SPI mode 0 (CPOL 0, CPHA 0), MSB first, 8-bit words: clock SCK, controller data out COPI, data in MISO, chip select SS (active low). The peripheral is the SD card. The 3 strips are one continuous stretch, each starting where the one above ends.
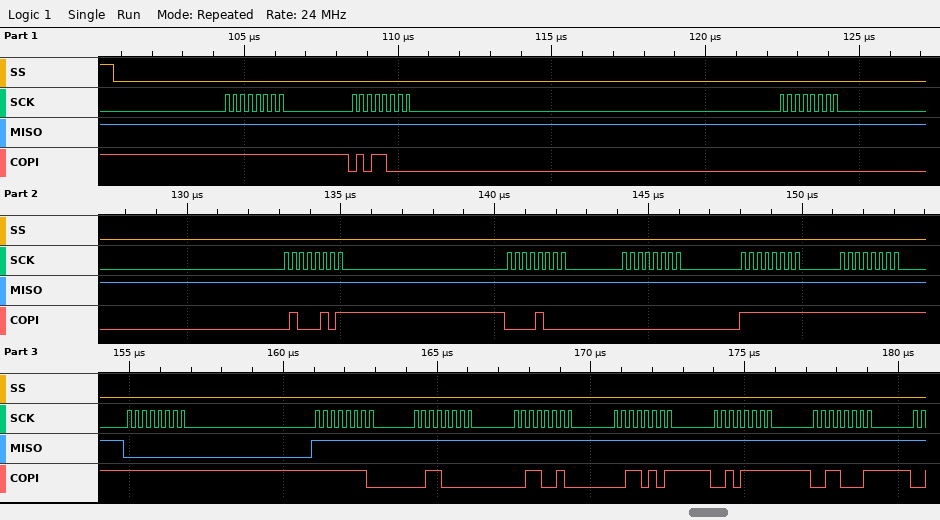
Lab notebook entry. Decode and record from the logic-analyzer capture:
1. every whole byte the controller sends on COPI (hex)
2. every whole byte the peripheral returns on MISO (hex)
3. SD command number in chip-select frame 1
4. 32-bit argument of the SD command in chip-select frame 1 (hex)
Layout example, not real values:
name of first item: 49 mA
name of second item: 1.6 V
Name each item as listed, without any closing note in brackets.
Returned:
every whole byte the controller sends on COPI: FF 58 00 45 08 00 FF FF FF FE 30 32 35 2F 31
every whole byte the peripheral returns on MISO: FF FF FF FF FF FF FF FF 00 FF FF FF FF FF FF
SD command number in chip-select frame 1: CMD24
32-bit argument of the SD command in chip-select frame 1: 0x00450800
